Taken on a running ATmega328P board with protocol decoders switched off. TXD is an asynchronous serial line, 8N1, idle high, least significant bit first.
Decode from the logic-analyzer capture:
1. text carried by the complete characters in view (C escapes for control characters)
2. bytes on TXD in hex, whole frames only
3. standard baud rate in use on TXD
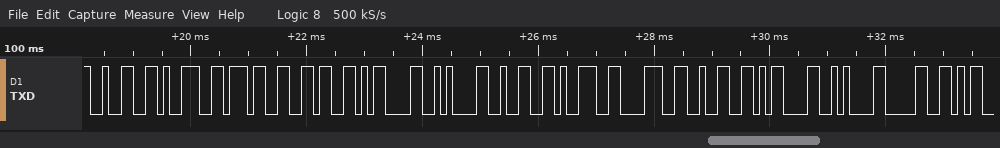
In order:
"2976\r\n2982\r\n0"
0x32 0x39 0x37 0x36 0x0D 0x0A 0x32 0x39 0x38 0x32 0x0D 0x0A 0x30
9600 baud
